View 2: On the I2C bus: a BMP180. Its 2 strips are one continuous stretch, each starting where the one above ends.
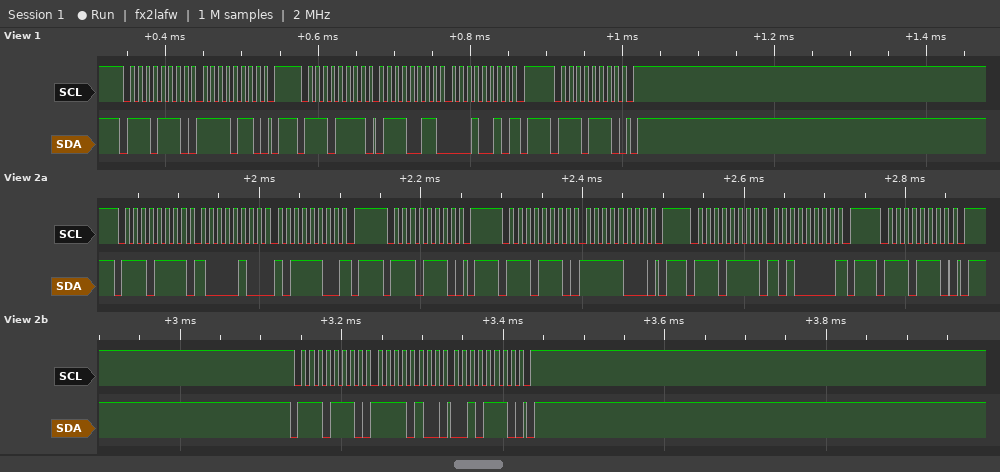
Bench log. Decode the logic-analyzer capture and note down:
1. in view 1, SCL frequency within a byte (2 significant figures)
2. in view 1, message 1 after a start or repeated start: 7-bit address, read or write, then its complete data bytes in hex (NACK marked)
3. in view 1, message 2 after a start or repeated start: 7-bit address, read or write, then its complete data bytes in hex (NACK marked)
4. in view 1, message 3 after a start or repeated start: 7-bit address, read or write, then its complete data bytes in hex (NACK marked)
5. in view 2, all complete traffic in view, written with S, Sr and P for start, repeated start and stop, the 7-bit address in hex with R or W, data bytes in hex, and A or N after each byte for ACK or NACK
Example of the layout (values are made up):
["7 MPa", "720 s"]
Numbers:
["100 kHz", "0x77 write: F6", "0x77 read: 73 12 NACK", "0x77 write", "S 77R A 84 A BC N P S 77W A P S 77W A F8 A P S 77R A A0 N P S 77W A P S 77W A F4 A 2E A P"]
